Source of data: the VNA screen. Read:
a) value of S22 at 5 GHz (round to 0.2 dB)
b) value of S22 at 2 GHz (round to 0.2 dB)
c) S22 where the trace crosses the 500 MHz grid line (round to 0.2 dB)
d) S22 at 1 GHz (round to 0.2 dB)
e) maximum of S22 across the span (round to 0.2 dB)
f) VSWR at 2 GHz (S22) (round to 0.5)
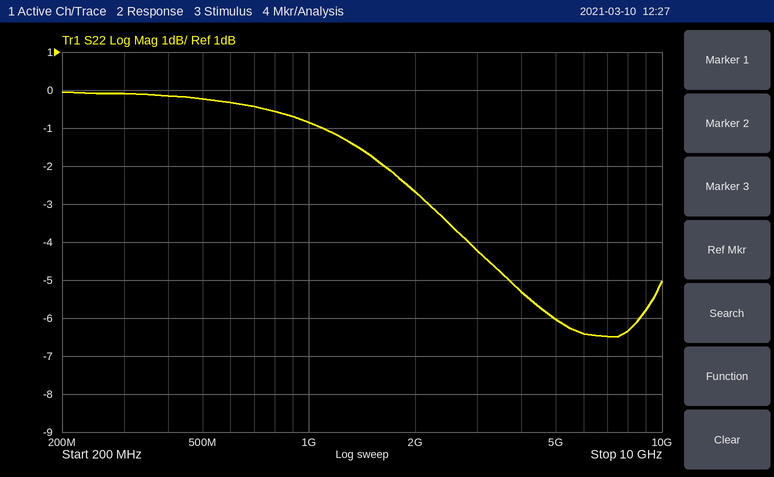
-6.0 dB
-2.6 dB
-0.2 dB
-0.8 dB
0.0 dB
6.5
